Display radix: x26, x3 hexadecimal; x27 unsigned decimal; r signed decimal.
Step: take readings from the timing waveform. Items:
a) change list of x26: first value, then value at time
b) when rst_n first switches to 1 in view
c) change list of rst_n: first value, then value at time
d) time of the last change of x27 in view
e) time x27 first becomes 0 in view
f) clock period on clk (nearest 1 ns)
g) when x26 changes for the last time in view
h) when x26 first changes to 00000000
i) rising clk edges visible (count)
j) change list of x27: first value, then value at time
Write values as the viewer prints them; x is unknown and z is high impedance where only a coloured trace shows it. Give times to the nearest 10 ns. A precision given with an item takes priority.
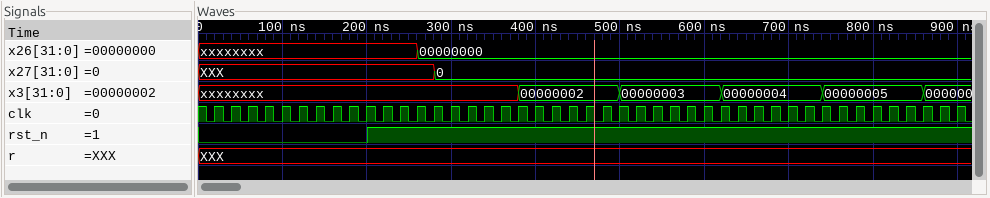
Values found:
xxxxxxxx, 00000000 at 260 ns
200 ns
0, 1 at 200 ns
280 ns
280 ns
20 ns
260 ns
260 ns
45
XXX, 0 at 280 ns
